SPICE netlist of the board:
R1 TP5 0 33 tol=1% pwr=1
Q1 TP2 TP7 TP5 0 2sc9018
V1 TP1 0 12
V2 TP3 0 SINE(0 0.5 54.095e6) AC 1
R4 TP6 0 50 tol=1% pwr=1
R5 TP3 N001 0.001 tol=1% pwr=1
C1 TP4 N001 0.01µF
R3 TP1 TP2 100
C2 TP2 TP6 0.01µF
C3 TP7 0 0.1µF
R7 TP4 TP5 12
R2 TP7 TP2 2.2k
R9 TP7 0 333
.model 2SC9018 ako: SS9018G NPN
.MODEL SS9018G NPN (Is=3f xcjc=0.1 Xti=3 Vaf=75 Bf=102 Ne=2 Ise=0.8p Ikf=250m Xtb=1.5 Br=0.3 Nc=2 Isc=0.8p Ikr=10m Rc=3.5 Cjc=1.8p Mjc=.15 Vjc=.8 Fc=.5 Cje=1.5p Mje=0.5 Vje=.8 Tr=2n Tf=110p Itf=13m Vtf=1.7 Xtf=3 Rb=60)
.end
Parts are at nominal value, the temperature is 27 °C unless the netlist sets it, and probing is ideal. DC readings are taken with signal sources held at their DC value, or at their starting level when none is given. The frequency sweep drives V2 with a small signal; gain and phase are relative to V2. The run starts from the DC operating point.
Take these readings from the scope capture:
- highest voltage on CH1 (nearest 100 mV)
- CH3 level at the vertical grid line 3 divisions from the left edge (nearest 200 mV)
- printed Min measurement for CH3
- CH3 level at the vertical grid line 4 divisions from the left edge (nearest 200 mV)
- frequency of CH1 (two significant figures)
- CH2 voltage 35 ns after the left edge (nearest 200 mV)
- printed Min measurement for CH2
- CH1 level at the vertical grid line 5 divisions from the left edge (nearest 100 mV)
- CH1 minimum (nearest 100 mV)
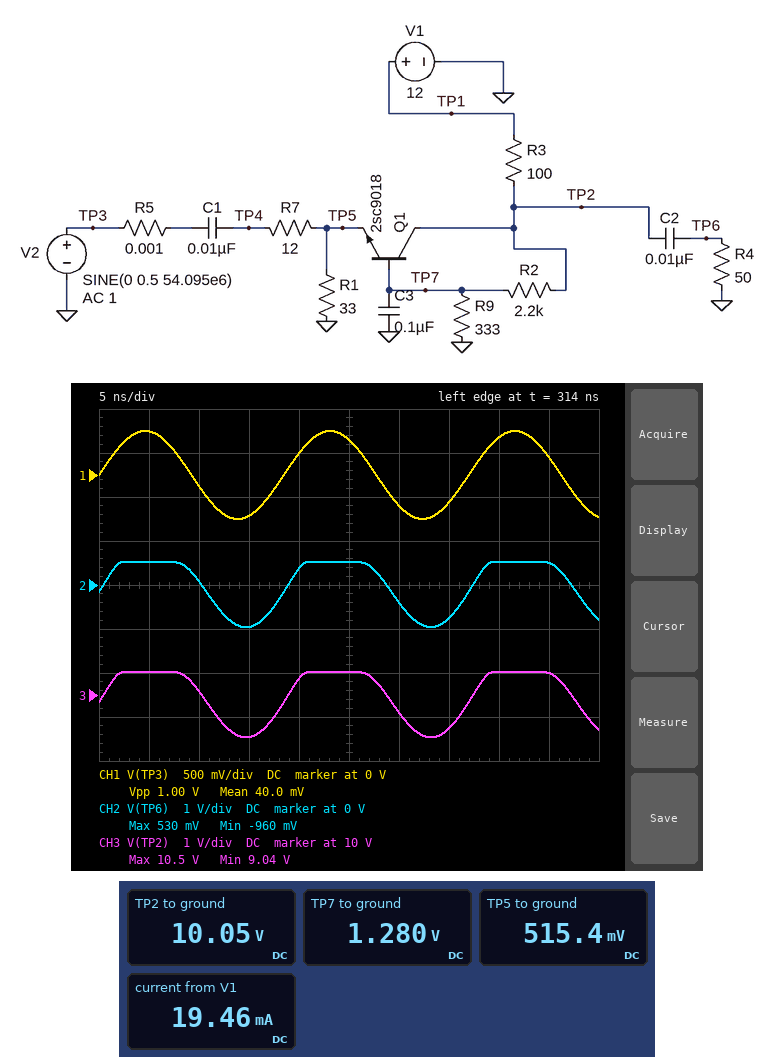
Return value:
500 mV
9.0 V
9.04 V
10.4 V
54 MHz
-800 mV
-960 mV
400 mV
-500 mV
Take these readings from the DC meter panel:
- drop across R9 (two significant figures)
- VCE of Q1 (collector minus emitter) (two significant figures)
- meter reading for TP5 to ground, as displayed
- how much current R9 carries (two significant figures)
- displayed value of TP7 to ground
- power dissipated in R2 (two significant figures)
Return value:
1.3 V
9.5 V
515.4 mV
3.8 mA
1.280 V
35 mW
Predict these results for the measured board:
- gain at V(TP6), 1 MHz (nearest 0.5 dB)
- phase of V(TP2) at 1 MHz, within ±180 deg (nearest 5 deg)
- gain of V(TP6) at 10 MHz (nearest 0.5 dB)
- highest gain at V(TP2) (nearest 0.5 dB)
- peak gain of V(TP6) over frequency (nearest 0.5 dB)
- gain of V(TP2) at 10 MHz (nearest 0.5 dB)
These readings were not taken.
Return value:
3.0 dB
35 deg
6.5 dB
6.5 dB
6.5 dB
6.5 dB
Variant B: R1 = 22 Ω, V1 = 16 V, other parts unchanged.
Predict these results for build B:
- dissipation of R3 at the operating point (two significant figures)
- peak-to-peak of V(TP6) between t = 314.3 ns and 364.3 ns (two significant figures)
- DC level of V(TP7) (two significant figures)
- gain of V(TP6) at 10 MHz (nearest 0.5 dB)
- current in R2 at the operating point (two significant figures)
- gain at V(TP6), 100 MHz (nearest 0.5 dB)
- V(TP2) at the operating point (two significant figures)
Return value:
140 mW
2.1 V
1.5 V
7.0 dB
4.9 mA
6.0 dB
12 V
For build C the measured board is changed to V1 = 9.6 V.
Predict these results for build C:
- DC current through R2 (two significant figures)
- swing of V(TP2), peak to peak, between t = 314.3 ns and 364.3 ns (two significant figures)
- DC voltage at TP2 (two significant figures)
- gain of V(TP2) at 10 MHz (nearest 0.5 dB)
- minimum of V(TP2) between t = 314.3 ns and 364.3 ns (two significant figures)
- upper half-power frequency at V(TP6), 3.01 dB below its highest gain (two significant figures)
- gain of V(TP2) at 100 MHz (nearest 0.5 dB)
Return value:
3.3 mA
1.2 V
8.3 V
6.0 dB
7.4 V
220 MHz
5.0 dB
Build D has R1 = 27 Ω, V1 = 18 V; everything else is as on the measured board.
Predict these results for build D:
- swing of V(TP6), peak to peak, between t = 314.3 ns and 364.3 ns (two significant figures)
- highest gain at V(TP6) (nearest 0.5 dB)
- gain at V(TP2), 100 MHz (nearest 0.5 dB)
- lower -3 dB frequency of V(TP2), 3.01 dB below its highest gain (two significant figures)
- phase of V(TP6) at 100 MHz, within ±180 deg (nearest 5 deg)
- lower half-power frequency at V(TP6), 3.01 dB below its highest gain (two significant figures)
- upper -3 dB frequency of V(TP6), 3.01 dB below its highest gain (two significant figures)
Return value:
2.1 V
7.0 dB
6.0 dB
1.1 MHz
-30 deg
1.2 MHz
190 MHz
